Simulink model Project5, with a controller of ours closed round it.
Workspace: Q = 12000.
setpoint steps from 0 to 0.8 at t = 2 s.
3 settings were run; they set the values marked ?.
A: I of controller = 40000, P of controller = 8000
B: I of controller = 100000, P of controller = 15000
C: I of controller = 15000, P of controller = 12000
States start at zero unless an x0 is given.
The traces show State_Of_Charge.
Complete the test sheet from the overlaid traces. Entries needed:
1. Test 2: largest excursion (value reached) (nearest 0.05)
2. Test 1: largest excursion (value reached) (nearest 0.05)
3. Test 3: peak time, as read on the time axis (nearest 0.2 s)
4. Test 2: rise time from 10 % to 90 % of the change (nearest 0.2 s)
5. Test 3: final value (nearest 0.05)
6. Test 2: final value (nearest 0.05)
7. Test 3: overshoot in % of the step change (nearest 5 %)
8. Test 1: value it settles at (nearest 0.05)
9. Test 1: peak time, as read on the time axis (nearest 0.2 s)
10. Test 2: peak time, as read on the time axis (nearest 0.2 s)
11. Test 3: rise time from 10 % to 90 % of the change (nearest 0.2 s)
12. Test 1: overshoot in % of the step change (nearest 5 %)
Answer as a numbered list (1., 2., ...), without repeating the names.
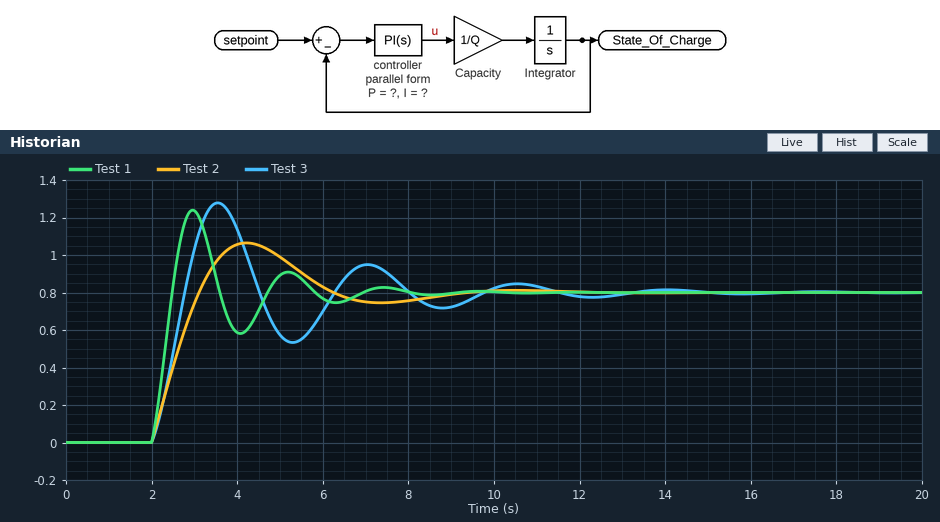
1. 1.05
2. 1.25
3. 3.6 s
4. 0.8 s
5. 0.80
6. 0.80
7. 60 %
8. 0.80
9. 3.0 s
10. 4.2 s
11. 0.6 s
12. 55 %
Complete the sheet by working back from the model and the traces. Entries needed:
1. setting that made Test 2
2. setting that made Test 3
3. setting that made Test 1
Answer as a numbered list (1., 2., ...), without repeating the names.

1. C
2. A
3. B
